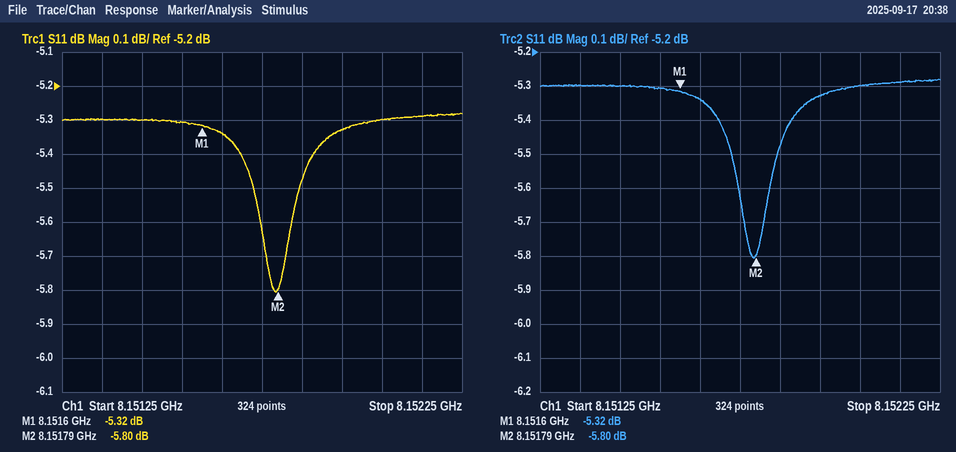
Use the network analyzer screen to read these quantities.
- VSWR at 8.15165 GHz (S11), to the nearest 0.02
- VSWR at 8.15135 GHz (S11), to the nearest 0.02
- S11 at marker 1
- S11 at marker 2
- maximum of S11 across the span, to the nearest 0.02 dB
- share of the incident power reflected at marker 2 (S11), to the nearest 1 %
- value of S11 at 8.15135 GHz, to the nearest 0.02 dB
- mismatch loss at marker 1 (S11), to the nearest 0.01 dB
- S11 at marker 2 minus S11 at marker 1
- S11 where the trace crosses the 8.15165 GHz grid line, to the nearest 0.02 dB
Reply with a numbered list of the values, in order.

1. 3.36
2. 3.38
3. -5.32 dB
4. -5.80 dB
5. -5.28 dB
6. 26 %
7. -5.30 dB
8. 1.51 dB
9. -0.48 dB
10. -5.34 dB
